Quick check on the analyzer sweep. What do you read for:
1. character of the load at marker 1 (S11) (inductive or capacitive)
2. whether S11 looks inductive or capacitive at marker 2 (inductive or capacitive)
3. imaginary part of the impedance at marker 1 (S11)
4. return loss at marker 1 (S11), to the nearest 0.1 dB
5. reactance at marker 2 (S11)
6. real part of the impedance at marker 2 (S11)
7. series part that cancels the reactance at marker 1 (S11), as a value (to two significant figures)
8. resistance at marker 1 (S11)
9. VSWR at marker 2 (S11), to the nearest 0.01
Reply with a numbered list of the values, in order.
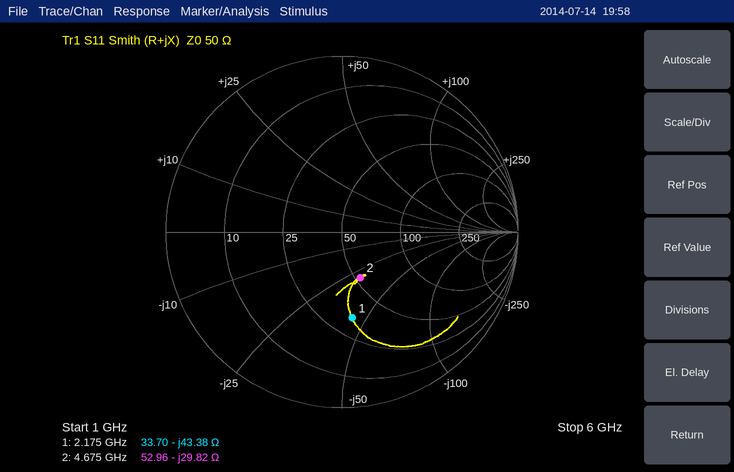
1. capacitive
2. capacitive
3. -43.38 Ω
4. 6.2 dB
5. -29.82 Ω
6. 52.96 Ω
7. 3.2 nH
8. 33.70 Ω
9. 1.78
